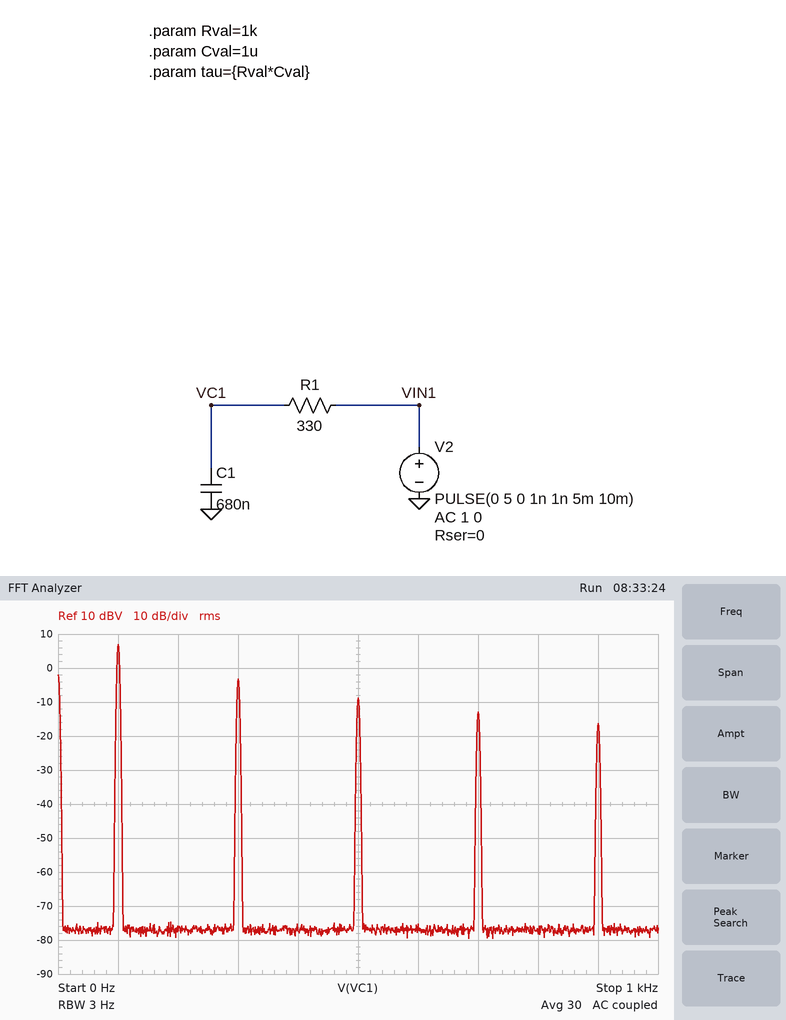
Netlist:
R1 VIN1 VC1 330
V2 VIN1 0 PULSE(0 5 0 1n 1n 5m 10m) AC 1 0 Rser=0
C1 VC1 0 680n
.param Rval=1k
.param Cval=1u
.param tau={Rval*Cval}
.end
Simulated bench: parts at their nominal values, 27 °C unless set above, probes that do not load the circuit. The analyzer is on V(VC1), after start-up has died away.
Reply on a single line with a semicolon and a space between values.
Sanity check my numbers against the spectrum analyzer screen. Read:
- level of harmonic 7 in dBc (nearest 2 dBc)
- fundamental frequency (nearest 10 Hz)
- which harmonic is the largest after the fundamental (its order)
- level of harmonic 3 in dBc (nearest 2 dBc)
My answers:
-20 dBc; 100 Hz; 3; -10 dBc
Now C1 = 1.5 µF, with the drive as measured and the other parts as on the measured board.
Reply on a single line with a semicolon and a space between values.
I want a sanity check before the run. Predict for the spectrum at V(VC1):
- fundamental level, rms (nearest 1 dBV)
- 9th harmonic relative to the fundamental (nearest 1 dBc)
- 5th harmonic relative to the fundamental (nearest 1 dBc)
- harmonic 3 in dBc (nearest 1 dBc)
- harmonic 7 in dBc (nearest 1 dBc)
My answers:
7 dBV; -28 dBc; -19 dBc; -12 dBc; -24 dBc
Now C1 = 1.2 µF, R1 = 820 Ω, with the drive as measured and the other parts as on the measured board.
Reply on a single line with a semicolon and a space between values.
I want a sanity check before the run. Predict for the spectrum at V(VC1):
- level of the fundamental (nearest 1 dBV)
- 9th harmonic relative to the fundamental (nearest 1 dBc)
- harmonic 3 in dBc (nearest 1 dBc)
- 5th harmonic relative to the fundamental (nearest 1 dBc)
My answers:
6 dBV; -33 dBc; -15 dBc; -23 dBc
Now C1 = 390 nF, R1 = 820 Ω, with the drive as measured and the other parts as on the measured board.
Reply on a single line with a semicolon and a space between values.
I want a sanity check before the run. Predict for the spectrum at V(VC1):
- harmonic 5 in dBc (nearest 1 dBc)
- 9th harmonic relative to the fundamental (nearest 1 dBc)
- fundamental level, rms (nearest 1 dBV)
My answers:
-17 dBc; -25 dBc; 7 dBV
